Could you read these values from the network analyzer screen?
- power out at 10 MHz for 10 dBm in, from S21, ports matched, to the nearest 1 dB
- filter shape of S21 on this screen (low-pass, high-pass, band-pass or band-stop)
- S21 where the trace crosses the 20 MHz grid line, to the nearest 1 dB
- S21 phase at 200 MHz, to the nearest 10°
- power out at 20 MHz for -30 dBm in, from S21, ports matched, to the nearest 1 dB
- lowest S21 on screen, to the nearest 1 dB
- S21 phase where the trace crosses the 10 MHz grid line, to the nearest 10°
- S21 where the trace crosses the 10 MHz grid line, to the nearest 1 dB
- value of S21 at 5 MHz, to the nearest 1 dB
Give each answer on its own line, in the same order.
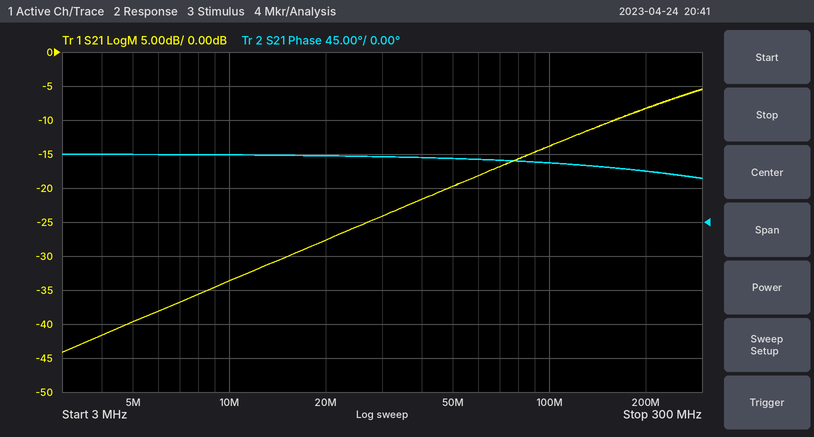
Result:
-24 dBm
high-pass
-28 dB
70°
-58 dBm
-44 dB
90°
-34 dB
-40 dB
